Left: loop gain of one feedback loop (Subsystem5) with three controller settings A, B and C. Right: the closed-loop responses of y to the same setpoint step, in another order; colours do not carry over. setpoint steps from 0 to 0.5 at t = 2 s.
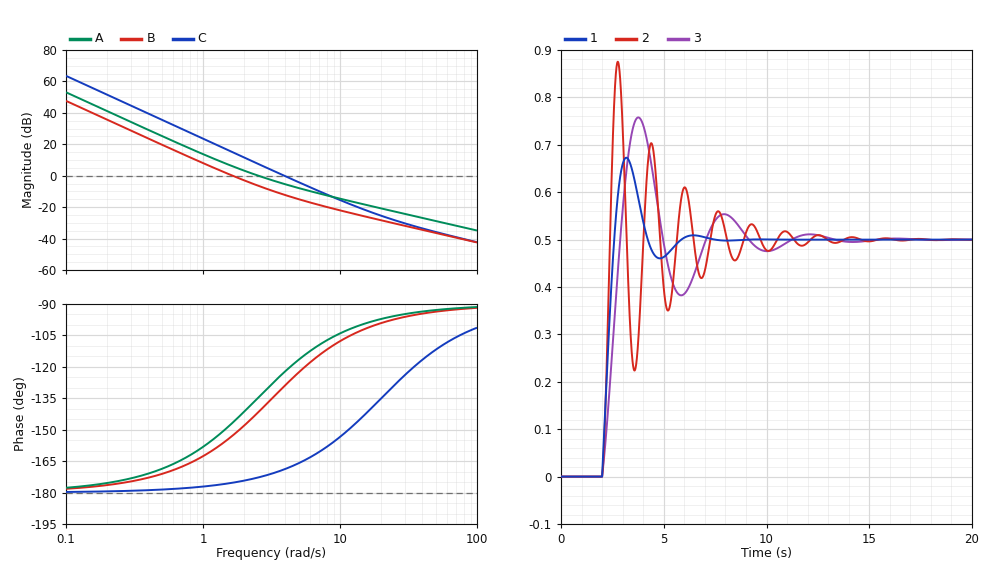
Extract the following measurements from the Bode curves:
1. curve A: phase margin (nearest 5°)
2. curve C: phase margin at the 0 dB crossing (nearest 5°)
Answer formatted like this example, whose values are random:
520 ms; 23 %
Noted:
45°; 10°
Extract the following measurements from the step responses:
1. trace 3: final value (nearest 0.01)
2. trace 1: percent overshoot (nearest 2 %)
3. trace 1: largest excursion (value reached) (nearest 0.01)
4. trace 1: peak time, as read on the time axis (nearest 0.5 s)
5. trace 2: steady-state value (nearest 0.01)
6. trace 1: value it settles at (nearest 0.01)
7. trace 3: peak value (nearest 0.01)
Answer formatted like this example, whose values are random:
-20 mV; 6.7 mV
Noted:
0.50; 34 %; 0.67; 3.0 s; 0.50; 0.50; 0.76
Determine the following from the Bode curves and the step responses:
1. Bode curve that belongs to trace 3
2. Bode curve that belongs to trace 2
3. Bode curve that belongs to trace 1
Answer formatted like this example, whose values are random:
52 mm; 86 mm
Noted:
B; C; A
